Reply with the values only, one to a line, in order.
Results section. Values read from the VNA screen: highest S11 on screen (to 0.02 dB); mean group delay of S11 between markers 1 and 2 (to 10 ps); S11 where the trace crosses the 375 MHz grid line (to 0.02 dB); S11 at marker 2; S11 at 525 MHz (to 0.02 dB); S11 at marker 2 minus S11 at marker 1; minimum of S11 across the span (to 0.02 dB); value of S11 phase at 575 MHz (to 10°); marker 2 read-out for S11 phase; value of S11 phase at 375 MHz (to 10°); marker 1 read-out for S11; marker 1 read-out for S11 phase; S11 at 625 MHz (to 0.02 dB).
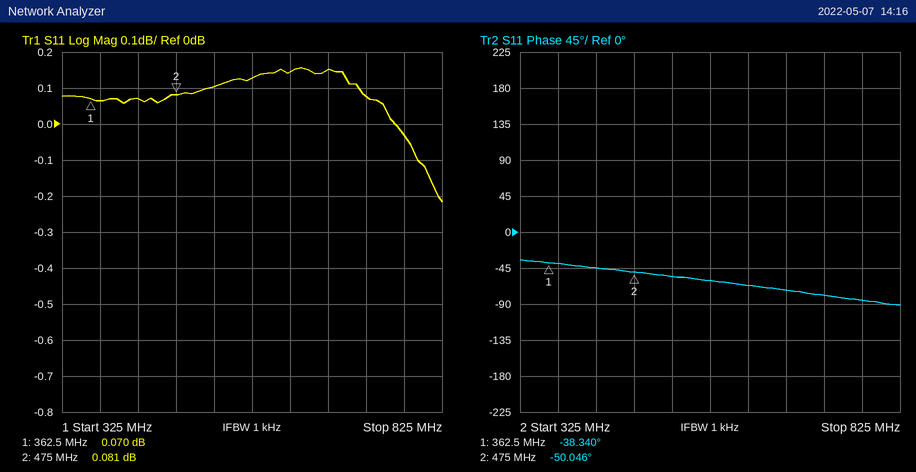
0.16 dB
290 ps
0.06 dB
0.081 dB
0.10 dB
0.011 dB
-0.22 dB
-60°
-50.046°
-40°
0.070 dB
-38.340°
0.14 dB
